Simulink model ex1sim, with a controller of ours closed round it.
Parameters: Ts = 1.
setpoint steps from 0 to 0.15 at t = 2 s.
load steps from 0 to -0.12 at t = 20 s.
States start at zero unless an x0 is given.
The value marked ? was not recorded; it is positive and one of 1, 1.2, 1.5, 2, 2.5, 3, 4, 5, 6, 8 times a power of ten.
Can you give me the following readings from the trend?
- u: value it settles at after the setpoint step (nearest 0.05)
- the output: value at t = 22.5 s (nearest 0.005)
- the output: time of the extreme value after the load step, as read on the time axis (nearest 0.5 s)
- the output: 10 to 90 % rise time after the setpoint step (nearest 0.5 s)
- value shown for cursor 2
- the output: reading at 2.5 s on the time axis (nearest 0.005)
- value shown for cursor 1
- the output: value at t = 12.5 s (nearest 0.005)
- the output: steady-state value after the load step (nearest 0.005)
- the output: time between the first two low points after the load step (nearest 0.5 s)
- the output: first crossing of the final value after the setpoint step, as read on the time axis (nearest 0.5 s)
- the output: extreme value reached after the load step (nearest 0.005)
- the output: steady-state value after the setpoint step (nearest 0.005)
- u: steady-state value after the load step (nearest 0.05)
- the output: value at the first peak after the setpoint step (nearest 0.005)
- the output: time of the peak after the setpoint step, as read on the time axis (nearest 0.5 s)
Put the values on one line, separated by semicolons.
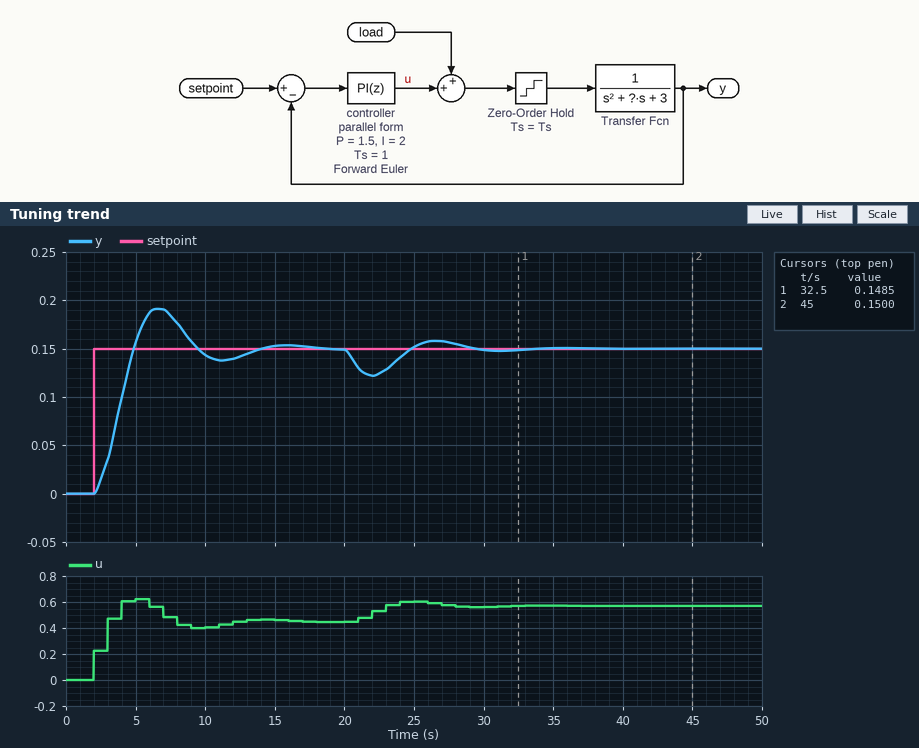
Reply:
0.45; 0.125; 22.0 s; 2.0 s; 0.1500; 0.015; 0.1485; 0.140; 0.150; 9.0 s; 5.0 s; 0.120; 0.150; 0.55; 0.190; 6.5 s
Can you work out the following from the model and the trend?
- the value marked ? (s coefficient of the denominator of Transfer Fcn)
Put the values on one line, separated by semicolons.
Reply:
4
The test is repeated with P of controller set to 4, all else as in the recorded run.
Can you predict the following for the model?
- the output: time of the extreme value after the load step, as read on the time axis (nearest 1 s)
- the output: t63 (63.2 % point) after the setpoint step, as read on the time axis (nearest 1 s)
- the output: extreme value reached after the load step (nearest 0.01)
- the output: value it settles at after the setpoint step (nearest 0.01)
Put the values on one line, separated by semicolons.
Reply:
21 s; 3 s; 0.13; 0.15
